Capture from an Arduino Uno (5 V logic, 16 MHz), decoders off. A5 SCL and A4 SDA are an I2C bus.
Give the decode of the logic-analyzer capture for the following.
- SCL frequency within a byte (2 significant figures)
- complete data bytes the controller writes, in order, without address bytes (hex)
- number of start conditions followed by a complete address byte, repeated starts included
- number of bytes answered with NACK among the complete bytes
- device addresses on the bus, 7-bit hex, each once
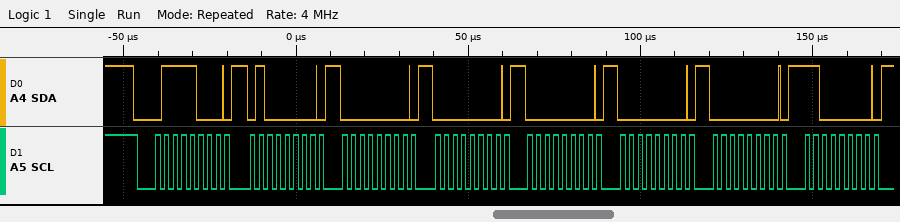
400 kHz
40 00 00 00 00 00 C0
1
0
0x3C
